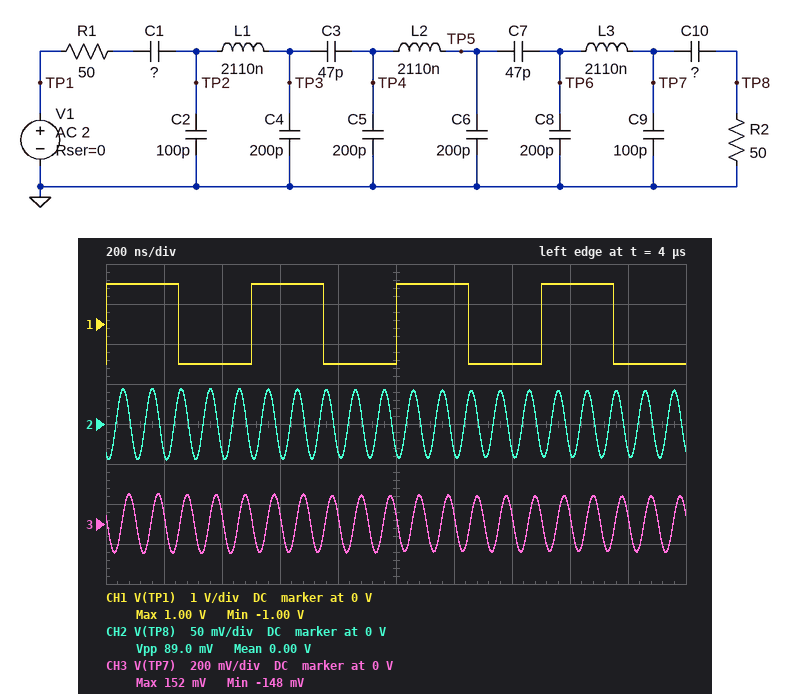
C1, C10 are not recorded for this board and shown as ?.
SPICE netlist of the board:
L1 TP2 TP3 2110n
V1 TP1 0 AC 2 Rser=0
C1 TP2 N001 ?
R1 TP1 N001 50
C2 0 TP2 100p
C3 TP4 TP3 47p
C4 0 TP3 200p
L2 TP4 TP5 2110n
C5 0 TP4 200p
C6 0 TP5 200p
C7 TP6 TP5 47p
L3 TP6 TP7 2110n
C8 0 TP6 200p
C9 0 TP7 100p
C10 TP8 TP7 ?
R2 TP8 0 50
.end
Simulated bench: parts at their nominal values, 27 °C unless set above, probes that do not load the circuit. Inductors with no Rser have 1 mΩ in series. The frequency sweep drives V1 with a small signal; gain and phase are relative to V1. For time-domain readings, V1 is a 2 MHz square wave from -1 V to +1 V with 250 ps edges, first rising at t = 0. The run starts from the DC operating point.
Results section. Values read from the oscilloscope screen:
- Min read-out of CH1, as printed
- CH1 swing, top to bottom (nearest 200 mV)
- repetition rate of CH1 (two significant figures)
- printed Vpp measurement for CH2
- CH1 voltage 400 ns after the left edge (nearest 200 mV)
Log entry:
-1.00 V
2.0 V
2.0 MHz
89.0 mV
-1.0 V
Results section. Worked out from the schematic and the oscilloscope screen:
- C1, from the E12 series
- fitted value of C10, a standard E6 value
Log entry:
56 pF
100 pF
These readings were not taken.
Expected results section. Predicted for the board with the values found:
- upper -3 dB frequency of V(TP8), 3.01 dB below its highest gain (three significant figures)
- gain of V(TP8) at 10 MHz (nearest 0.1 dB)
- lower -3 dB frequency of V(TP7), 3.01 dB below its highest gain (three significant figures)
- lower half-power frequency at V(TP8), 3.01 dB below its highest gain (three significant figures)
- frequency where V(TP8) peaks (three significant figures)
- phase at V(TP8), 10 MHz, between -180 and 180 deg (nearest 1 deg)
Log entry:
9.82 MHz
-15.3 dB
9.60 MHz
9.60 MHz
9.70 MHz
-122 deg
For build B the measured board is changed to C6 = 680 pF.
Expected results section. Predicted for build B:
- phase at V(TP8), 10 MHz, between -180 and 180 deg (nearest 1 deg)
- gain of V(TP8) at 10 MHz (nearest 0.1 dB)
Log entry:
-154 deg
-37.2 dB
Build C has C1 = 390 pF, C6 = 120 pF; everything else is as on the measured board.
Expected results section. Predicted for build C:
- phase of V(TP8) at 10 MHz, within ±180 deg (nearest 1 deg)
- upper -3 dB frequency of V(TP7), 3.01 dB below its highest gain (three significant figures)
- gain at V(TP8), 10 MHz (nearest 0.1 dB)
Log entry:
-129 deg
11.8 MHz
-13.6 dB
